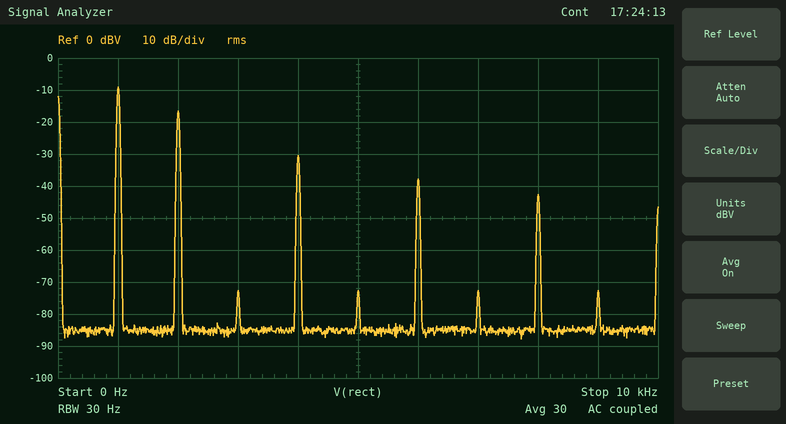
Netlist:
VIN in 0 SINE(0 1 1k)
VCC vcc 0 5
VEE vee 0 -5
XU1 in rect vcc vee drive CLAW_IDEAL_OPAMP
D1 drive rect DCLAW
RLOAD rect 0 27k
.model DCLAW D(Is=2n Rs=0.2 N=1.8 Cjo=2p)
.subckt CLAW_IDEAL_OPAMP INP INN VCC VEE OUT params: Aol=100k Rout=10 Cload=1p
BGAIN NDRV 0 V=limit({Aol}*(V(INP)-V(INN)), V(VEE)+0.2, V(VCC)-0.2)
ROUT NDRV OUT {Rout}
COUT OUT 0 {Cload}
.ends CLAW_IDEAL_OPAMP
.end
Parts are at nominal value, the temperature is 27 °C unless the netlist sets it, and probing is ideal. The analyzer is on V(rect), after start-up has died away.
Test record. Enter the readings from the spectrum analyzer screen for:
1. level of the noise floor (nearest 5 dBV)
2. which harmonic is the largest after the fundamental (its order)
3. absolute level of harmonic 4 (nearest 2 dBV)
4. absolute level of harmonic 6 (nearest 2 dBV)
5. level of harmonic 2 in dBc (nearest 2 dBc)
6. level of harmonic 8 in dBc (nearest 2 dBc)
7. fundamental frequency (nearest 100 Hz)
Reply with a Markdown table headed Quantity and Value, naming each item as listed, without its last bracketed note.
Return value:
| Quantity | Value |
|---|---|
| level of the noise floor | -85 dBV |
| which harmonic is the largest after the fundamental | 2 |
| absolute level of harmonic 4 | -30 dBV |
| absolute level of harmonic 6 | -38 dBV |
| level of harmonic 2 in dBc | -8 dBc |
| level of harmonic 8 in dBc | -34 dBc |
| fundamental frequency | 1.0 kHz |
